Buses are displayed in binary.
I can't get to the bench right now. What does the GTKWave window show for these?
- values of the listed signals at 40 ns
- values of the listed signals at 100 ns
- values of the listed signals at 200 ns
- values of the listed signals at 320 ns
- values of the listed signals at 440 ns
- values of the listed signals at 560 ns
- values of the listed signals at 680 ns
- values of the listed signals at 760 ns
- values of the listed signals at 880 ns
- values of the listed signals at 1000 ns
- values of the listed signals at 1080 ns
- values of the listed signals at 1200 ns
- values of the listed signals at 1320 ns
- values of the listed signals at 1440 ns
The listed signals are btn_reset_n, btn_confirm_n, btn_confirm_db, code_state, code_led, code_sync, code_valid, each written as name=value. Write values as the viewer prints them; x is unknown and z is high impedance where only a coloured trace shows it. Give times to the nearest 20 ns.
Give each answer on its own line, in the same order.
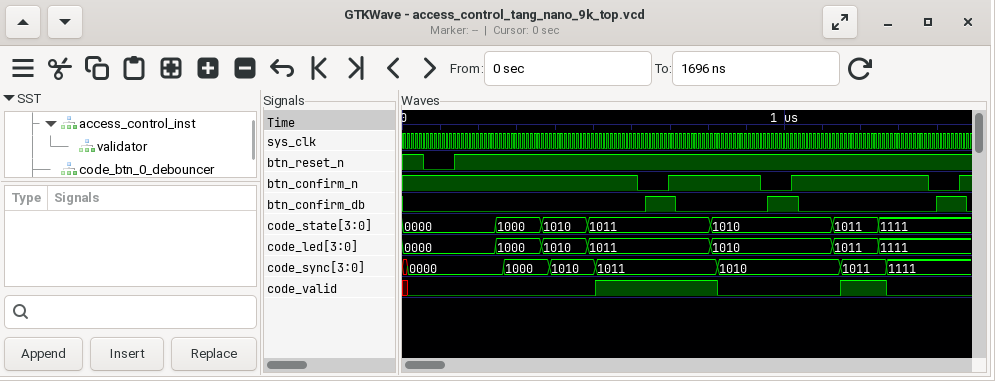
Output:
btn_reset_n=1, btn_confirm_n=1, btn_confirm_db=0, code_state=0000, code_led=0000, code_sync=0000, code_valid=0
btn_reset_n=0, btn_confirm_n=1, btn_confirm_db=0, code_state=0000, code_led=0000, code_sync=0000, code_valid=0
btn_reset_n=1, btn_confirm_n=1, btn_confirm_db=0, code_state=0000, code_led=0000, code_sync=0000, code_valid=0
btn_reset_n=1, btn_confirm_n=1, btn_confirm_db=0, code_state=1000, code_led=1000, code_sync=1000, code_valid=0
btn_reset_n=1, btn_confirm_n=1, btn_confirm_db=0, code_state=1010, code_led=1010, code_sync=1010, code_valid=0
btn_reset_n=1, btn_confirm_n=1, btn_confirm_db=0, code_state=1011, code_led=1011, code_sync=1011, code_valid=1
btn_reset_n=1, btn_confirm_n=0, btn_confirm_db=1, code_state=1011, code_led=1011, code_sync=1011, code_valid=1
btn_reset_n=1, btn_confirm_n=1, btn_confirm_db=0, code_state=1011, code_led=1011, code_sync=1011, code_valid=1
btn_reset_n=1, btn_confirm_n=1, btn_confirm_db=0, code_state=1010, code_led=1010, code_sync=1010, code_valid=0
btn_reset_n=1, btn_confirm_n=0, btn_confirm_db=1, code_state=1010, code_led=1010, code_sync=1010, code_valid=0
btn_reset_n=1, btn_confirm_n=1, btn_confirm_db=0, code_state=1010, code_led=1010, code_sync=1010, code_valid=0
btn_reset_n=1, btn_confirm_n=1, btn_confirm_db=0, code_state=1011, code_led=1011, code_sync=1011, code_valid=1
btn_reset_n=1, btn_confirm_n=1, btn_confirm_db=0, code_state=1111, code_led=1111, code_sync=1111, code_valid=0
btn_reset_n=1, btn_confirm_n=0, btn_confirm_db=1, code_state=1111, code_led=1111, code_sync=1111, code_valid=0
